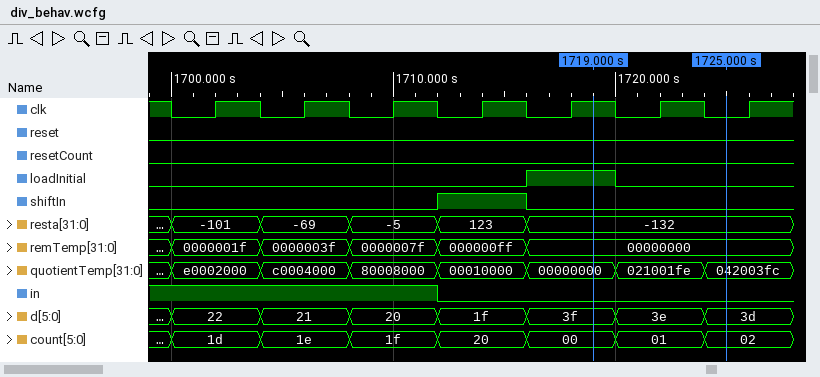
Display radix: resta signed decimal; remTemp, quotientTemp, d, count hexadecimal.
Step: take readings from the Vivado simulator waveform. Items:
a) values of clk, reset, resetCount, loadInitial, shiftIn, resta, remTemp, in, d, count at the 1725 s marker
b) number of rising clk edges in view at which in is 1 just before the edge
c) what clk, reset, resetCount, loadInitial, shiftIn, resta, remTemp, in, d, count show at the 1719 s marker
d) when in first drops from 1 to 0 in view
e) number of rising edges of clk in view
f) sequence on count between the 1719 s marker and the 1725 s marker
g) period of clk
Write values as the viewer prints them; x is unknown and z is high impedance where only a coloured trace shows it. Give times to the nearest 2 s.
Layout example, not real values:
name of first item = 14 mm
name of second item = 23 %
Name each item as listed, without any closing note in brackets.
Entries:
values of clk, reset, resetCount, loadInitial, shiftIn, resta, remTemp, in, d, count at the 1725 s marker = clk=0, reset=0, resetCount=0, loadInitial=0, shiftIn=0, resta=-132, remTemp=00000000, in=0, d=3d, count=02
number of rising clk edges in view at which in is 1 just before the edge = 3
what clk, reset, resetCount, loadInitial, shiftIn, resta, remTemp, in, d, count show at the 1719 s marker = clk=1, reset=0, resetCount=0, loadInitial=1, shiftIn=0, resta=-132, remTemp=00000000, in=0, d=3f, count=00
when in first drops from 1 to 0 in view = 1712 s
number of rising edges of clk in view = 7
sequence on count between the 1719 s marker and the 1725 s marker = 00, 01, 02
period of clk = 4 s
